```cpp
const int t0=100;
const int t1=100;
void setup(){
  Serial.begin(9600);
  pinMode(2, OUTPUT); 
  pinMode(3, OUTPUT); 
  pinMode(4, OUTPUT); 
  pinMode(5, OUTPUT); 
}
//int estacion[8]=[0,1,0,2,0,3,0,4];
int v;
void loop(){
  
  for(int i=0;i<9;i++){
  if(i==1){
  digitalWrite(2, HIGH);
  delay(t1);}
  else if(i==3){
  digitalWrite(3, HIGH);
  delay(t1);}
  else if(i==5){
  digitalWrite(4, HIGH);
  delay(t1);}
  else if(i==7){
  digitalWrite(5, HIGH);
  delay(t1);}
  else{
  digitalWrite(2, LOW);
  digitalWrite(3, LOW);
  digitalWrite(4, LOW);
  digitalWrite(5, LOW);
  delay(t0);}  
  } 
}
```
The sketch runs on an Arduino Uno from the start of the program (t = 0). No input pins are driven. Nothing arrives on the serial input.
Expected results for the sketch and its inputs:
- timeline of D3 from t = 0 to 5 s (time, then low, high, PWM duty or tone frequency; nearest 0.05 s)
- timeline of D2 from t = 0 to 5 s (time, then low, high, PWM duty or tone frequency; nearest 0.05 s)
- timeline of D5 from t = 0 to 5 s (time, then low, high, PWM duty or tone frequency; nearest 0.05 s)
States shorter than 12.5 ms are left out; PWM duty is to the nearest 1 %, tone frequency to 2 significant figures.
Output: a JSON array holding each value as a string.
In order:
["0 s low; 0.3 s high; 0.4 s low; 1.2 s high; 1.3 s low; 2.1 s high; 2.2 s low; 3 s high; 3.1 s low; 3.9 s high; 4 s low; 4.8 s high; 4.9 s low", "0 s low; 0.1 s high; 0.2 s low; 1 s high; 1.1 s low; 1.9 s high; 2 s low; 2.8 s high; 2.9 s low; 3.7 s high; 3.8 s low; 4.6 s high; 4.7 s low", "0 s low; 0.7 s high; 0.8 s low; 1.6 s high; 1.7 s low; 2.5 s high; 2.6 s low; 3.4 s high; 3.5 s low; 4.3 s high; 4.4 s low"]
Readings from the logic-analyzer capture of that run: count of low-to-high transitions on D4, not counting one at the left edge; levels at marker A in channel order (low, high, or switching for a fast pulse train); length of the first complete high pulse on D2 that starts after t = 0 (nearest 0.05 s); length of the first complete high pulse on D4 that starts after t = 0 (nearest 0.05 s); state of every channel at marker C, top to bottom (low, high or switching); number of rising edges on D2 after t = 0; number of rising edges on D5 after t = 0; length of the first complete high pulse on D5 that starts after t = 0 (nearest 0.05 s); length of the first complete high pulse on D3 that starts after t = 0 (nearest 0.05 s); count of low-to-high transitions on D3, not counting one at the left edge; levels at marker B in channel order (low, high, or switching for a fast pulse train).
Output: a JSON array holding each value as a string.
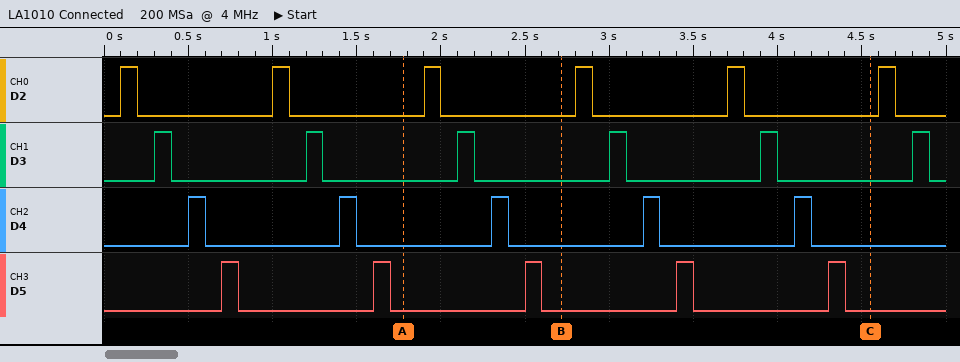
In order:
["5", "D2 low, D3 low, D4 low, D5 low", "0.10 s", "0.10 s", "D2 low, D3 low, D4 low, D5 low", "6", "5", "0.10 s", "0.10 s", "6", "D2 low, D3 low, D4 low, D5 low"]
